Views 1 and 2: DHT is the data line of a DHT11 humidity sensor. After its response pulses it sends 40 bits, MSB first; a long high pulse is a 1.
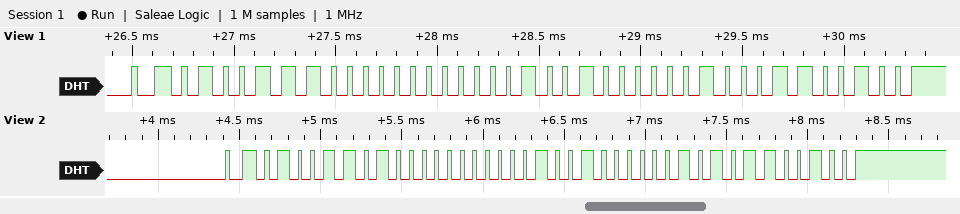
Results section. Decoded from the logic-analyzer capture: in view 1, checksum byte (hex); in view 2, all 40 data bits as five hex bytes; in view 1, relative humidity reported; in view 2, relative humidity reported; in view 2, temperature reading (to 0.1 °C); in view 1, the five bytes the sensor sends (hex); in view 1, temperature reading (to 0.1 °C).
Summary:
0x64
4D 00 12 05 64
78 %
77 %
18.5 °C
4E 00 12 04 64
18.4 °C
